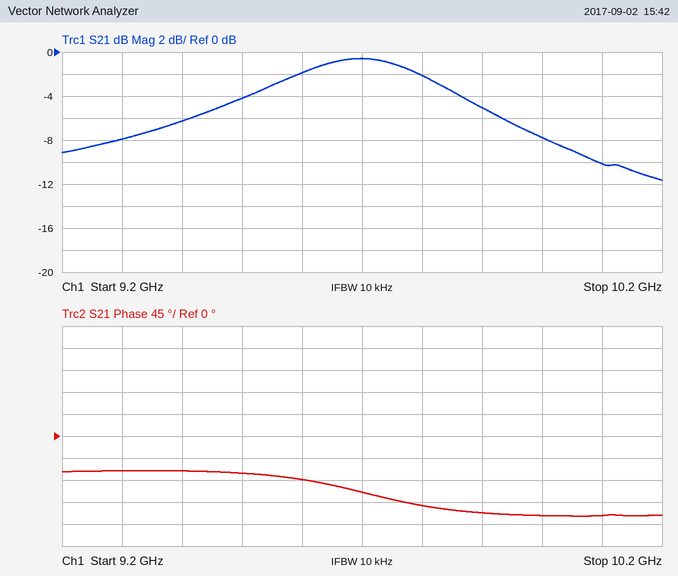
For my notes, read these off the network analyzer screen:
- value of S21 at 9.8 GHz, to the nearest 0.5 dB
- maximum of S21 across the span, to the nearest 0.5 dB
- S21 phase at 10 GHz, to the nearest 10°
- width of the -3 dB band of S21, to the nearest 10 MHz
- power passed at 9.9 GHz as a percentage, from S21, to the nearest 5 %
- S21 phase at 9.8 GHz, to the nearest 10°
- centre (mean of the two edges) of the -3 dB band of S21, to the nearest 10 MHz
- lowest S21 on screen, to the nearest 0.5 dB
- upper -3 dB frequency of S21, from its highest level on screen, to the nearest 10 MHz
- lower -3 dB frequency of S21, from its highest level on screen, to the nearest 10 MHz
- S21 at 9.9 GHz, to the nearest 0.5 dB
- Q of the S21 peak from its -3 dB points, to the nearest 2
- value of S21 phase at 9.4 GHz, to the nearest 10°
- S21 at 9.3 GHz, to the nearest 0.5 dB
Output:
-2.0 dB
-0.5 dB
-160°
320 MHz
30 %
-140°
9.69 GHz
-11.5 dB
9.85 GHz
9.53 GHz
-5.0 dB
30
-70°
-8.0 dB
